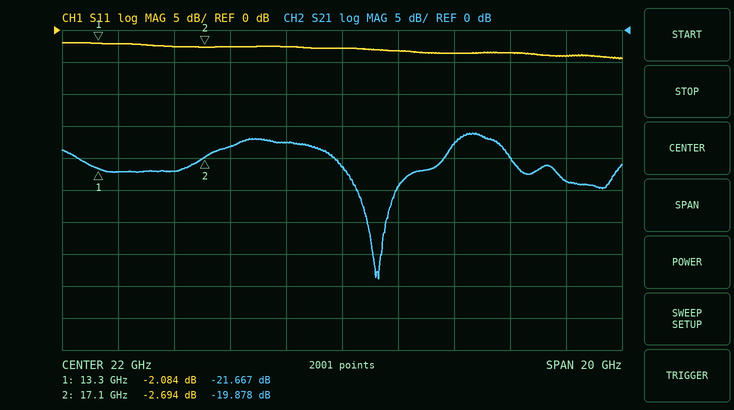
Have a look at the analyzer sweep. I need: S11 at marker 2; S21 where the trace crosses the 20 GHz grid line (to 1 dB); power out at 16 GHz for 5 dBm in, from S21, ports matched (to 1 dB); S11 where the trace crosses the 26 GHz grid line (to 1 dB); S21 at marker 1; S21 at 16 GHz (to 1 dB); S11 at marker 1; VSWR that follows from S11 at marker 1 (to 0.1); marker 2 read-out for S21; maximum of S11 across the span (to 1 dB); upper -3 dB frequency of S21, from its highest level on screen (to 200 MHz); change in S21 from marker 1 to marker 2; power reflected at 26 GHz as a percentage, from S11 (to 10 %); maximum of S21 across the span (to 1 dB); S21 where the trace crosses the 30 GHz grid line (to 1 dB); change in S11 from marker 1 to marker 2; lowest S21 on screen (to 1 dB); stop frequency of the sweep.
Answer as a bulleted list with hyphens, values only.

- -2.694 dB
- -18 dB
- -17 dBm
- -4 dB
- -21.667 dB
- -22 dB
- -2.084 dB
- 8.4
- -19.878 dB
- -2 dB
- 27.8 GHz
- 1.789 dB
- 40 %
- -16 dB
- -24 dB
- -0.610 dB
- -39 dB
- 32 GHz
